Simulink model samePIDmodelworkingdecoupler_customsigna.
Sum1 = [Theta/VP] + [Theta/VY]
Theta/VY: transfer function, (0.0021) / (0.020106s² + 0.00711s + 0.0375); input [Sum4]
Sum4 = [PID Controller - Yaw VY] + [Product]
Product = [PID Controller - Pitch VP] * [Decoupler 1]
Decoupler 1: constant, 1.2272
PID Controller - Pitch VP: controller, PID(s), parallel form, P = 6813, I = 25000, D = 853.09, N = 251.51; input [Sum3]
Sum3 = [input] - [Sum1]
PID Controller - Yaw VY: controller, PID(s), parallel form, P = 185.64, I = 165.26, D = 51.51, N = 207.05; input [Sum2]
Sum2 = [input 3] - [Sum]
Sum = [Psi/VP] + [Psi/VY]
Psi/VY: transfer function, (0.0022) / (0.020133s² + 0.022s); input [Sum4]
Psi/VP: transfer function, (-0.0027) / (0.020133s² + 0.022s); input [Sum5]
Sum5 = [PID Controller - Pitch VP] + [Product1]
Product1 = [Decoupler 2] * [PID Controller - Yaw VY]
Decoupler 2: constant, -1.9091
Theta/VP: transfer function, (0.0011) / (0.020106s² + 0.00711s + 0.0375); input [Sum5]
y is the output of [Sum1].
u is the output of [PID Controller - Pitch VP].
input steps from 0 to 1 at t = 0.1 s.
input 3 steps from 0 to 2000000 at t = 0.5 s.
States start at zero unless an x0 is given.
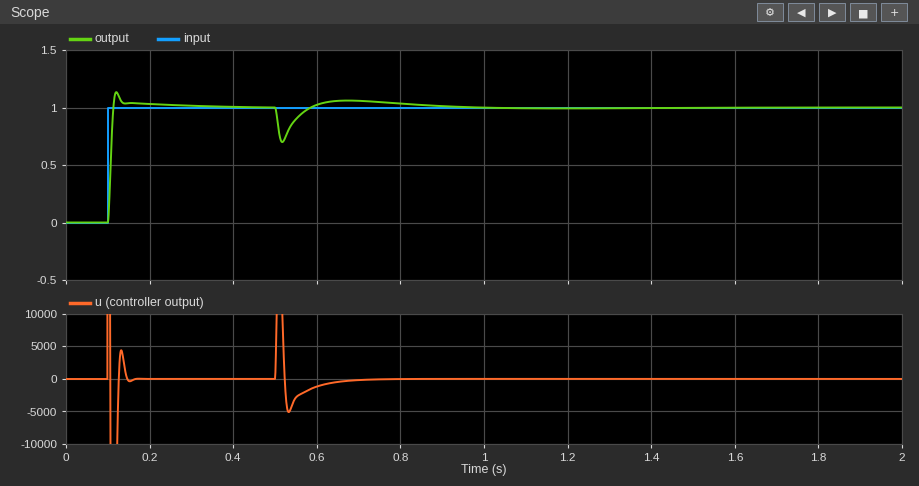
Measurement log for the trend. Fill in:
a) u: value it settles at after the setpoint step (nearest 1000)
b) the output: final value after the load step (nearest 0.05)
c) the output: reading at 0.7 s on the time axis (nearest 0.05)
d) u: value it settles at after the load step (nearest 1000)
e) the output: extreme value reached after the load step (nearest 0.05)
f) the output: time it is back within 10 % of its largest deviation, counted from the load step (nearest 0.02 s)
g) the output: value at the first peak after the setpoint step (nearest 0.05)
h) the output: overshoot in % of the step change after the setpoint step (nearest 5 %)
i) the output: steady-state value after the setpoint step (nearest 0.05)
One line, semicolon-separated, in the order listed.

0; 1.00; 1.05; 0; 0.70; 0.32 s; 1.15; 15 %; 1.00
